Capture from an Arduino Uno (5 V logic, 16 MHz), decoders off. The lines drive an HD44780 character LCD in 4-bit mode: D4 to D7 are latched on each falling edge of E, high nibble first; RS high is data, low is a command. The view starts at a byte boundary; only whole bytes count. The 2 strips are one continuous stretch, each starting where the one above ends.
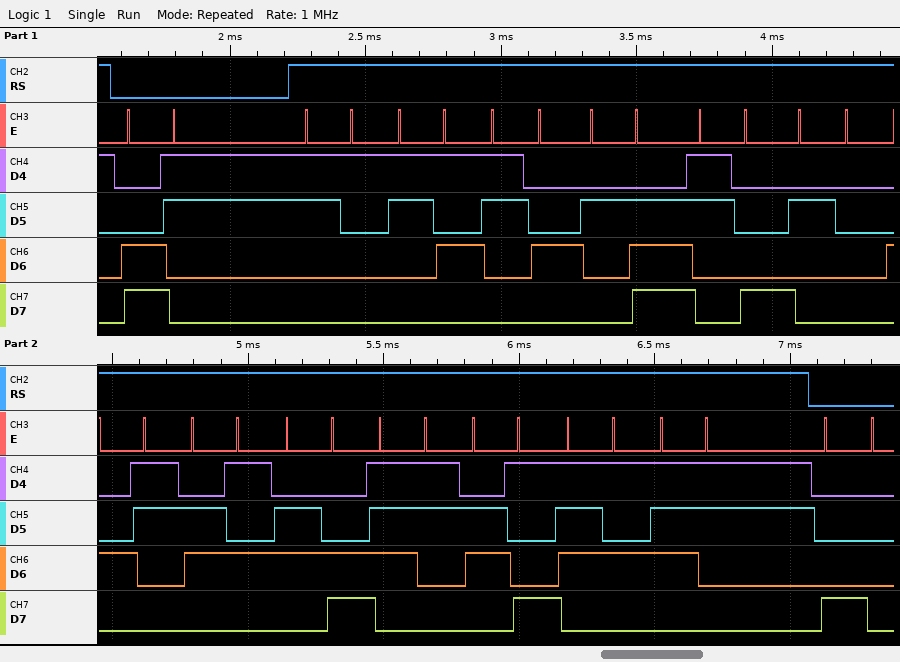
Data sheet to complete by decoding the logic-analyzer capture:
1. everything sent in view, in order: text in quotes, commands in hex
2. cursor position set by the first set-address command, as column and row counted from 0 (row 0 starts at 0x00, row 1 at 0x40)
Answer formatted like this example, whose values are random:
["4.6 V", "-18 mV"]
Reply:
["0xC3 \"154.8 Celsius\" 0x80", "column 3, row 1"]
